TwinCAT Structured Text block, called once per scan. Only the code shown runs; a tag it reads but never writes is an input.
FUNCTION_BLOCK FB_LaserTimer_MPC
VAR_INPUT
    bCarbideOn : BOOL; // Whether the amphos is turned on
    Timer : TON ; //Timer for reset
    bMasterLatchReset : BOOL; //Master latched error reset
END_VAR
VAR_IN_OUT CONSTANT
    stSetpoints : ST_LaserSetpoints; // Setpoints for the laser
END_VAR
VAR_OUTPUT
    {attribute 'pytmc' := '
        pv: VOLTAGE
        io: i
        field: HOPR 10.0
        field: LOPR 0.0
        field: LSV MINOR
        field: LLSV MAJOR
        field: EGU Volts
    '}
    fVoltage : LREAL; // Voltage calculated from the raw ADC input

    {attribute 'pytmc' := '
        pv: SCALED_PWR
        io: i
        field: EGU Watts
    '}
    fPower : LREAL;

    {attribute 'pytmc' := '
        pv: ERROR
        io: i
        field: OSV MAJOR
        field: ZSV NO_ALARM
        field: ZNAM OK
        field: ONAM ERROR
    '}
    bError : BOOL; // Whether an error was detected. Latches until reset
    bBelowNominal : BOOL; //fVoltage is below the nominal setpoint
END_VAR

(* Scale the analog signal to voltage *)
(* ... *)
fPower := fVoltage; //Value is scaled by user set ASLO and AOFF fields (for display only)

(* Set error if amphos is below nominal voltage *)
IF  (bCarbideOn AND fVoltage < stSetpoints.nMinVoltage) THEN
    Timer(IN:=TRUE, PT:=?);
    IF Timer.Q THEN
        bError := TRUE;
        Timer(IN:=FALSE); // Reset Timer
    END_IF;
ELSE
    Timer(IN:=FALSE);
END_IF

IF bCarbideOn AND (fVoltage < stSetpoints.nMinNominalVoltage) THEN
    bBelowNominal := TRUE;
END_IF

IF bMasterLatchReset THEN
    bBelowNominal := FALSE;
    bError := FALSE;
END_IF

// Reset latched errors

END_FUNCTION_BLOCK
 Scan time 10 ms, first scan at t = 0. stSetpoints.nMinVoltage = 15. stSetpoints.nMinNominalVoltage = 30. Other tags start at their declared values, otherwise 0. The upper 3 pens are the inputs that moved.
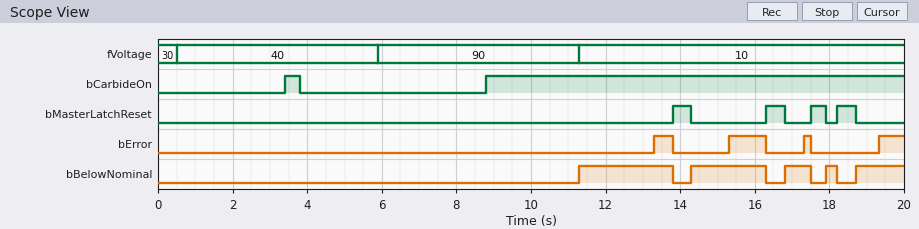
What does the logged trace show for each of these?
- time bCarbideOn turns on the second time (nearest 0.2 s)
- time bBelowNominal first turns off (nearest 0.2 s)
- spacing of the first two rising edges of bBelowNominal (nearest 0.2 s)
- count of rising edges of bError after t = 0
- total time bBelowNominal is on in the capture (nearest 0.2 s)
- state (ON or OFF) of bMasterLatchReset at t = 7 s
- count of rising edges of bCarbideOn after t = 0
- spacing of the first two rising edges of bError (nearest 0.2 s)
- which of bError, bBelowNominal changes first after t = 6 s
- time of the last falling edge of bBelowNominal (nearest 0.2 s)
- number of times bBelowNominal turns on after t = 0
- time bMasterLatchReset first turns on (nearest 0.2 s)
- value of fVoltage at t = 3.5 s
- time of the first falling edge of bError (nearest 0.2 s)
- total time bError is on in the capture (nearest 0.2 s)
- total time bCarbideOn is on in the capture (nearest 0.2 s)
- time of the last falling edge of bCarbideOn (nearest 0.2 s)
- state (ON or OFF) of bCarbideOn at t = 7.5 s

8.8 s
13.8 s
3.0 s
4
6.8 s
OFF
2
2.0 s
bBelowNominal
18.2 s
5
13.8 s
40
13.8 s
2.4 s
11.6 s
3.8 s
OFF
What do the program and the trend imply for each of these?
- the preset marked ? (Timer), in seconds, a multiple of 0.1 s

2.0 s
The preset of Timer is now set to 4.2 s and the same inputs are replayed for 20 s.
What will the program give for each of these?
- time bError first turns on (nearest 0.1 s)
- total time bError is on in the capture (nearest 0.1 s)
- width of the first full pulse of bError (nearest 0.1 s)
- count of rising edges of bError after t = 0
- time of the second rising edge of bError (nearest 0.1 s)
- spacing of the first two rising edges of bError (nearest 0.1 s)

15.5 s
1.1 s
0.8 s
2
19.7 s
4.2 s
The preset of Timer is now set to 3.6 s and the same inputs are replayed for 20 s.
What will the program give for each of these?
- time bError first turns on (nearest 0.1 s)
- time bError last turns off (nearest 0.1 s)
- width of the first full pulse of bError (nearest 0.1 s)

14.9 s
16.3 s
1.4 s
